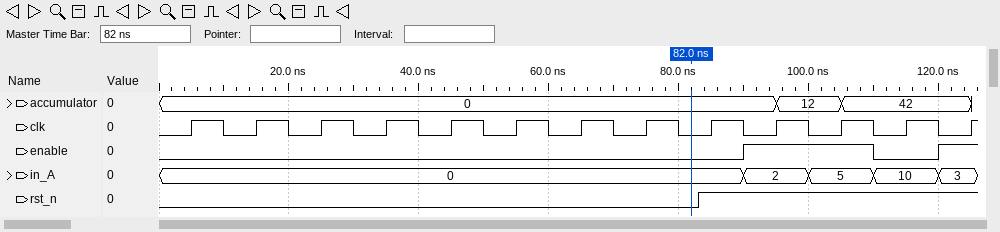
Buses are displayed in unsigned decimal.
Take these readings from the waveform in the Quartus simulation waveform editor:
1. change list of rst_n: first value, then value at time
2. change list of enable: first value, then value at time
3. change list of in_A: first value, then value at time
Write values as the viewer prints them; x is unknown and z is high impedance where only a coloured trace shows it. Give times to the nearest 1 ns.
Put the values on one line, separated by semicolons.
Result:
0, 1 at 83 ns; 0, 1 at 90 ns, 0 at 110 ns, 1 at 120 ns; 0, 2 at 90 ns, 5 at 100 ns, 10 at 110 ns, 3 at 120 ns
